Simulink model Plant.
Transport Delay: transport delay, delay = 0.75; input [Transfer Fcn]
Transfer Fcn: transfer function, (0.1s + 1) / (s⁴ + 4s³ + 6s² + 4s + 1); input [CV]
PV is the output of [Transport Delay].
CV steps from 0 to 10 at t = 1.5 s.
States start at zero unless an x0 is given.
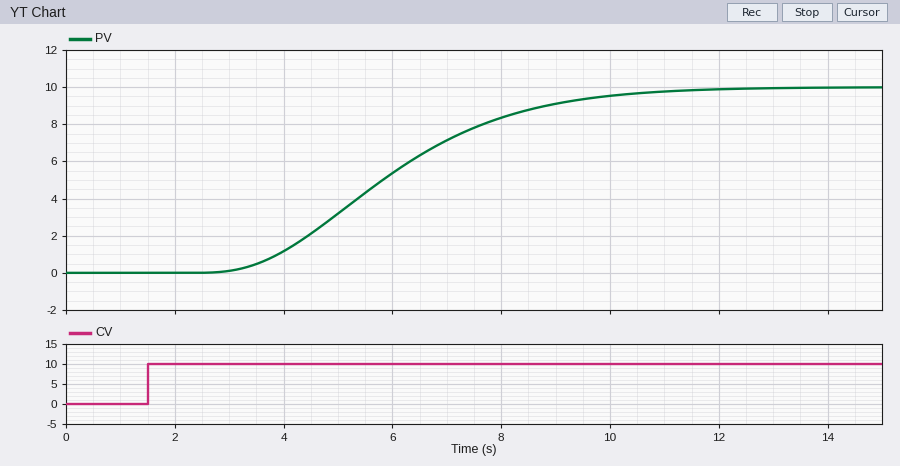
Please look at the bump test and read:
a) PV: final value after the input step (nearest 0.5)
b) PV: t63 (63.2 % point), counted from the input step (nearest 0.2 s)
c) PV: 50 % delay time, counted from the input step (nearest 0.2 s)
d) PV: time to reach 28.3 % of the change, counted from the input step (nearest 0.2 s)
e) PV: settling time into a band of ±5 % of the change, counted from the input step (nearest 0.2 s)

10.0
5.0 s
4.4 s
3.4 s
8.4 s
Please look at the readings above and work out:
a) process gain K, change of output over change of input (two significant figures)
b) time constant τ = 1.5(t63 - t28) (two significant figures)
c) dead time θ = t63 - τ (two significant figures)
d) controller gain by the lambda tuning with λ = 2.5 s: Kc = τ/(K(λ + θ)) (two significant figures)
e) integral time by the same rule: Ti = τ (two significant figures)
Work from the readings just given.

1.0
2.4 s
2.6 s
0.47
2.4 s
